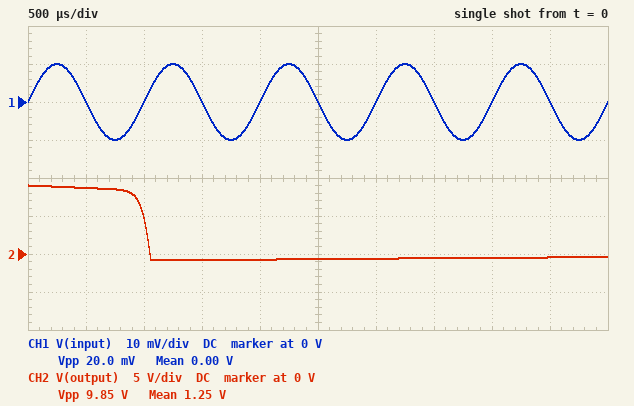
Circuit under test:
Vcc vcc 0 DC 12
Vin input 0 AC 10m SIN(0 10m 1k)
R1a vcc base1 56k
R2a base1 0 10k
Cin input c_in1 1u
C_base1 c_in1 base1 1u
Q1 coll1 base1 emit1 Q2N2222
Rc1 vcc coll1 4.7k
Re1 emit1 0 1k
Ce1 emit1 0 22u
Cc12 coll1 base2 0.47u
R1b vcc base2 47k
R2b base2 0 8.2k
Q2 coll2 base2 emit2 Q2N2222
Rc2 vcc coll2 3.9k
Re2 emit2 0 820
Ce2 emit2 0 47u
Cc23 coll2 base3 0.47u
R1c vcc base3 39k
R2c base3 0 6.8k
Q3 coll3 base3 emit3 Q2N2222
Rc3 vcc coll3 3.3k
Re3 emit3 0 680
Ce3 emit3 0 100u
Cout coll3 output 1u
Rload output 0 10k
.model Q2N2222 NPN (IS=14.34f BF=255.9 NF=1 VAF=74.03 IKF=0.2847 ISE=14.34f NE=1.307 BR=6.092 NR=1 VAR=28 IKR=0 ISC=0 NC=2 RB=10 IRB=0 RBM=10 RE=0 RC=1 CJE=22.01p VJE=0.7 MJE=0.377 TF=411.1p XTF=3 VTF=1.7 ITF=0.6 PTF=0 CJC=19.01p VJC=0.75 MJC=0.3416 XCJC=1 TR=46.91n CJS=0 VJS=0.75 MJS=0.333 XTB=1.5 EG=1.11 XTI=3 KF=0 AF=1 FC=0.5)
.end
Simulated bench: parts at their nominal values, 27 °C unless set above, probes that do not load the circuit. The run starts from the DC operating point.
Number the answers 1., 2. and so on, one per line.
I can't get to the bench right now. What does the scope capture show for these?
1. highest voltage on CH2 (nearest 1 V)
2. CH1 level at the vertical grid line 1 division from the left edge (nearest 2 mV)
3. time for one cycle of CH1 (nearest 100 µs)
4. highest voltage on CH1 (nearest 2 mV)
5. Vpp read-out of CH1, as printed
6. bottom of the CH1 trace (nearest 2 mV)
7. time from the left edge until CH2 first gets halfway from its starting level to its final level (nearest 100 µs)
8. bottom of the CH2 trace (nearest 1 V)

1. 9 V
2. 0 V
3. 1.0 ms
4. 10 mV
5. 20.0 mV
6. -10 mV
7. 1.0 ms
8. -1 V
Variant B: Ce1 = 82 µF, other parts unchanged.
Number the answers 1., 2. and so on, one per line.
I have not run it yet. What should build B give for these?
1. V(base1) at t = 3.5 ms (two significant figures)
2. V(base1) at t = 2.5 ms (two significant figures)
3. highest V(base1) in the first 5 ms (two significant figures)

1. 750 mV
2. 710 mV
3. 810 mV
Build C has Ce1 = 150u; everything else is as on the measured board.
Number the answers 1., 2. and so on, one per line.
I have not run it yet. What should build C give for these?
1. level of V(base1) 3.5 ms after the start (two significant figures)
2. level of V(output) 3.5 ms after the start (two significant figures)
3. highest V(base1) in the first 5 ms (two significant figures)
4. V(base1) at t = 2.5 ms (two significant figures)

1. 720 mV
2. -560 mV
3. 750 mV
4. 700 mV
